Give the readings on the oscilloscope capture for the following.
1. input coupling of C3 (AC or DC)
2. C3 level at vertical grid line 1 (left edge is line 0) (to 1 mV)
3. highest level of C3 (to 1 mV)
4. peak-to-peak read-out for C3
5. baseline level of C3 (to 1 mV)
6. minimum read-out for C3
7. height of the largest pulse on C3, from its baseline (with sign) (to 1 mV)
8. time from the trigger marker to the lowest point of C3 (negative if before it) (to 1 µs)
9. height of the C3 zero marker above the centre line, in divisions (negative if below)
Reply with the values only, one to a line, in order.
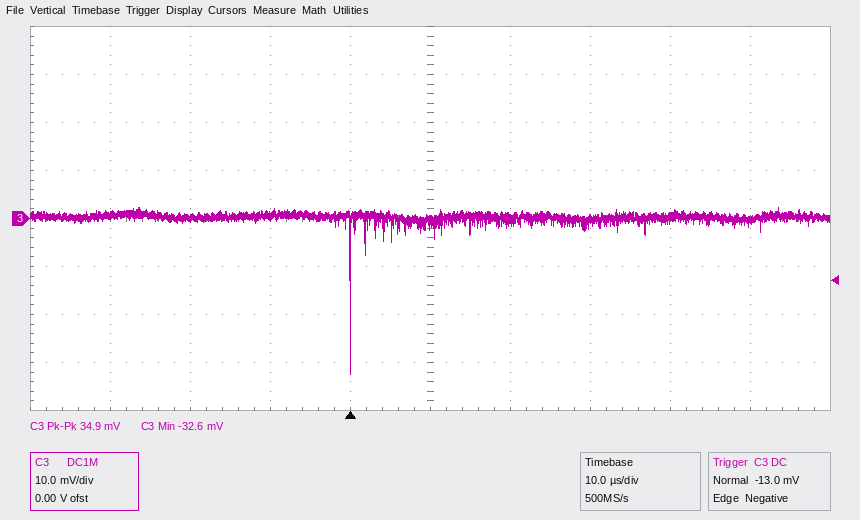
DC
1 mV
2 mV
34.9 mV
0 mV
-32.6 mV
-33 mV
0 µs
0.0 div
